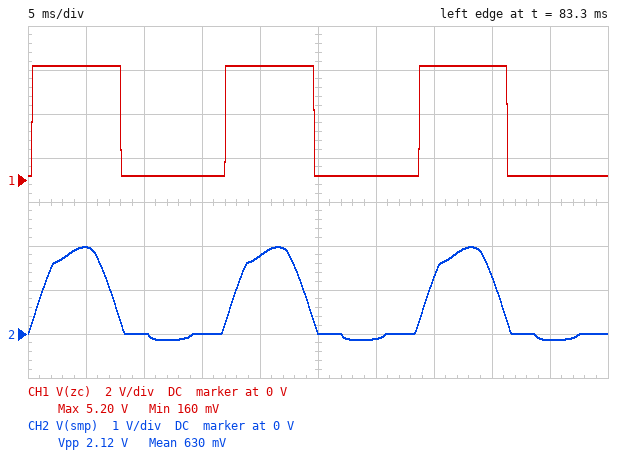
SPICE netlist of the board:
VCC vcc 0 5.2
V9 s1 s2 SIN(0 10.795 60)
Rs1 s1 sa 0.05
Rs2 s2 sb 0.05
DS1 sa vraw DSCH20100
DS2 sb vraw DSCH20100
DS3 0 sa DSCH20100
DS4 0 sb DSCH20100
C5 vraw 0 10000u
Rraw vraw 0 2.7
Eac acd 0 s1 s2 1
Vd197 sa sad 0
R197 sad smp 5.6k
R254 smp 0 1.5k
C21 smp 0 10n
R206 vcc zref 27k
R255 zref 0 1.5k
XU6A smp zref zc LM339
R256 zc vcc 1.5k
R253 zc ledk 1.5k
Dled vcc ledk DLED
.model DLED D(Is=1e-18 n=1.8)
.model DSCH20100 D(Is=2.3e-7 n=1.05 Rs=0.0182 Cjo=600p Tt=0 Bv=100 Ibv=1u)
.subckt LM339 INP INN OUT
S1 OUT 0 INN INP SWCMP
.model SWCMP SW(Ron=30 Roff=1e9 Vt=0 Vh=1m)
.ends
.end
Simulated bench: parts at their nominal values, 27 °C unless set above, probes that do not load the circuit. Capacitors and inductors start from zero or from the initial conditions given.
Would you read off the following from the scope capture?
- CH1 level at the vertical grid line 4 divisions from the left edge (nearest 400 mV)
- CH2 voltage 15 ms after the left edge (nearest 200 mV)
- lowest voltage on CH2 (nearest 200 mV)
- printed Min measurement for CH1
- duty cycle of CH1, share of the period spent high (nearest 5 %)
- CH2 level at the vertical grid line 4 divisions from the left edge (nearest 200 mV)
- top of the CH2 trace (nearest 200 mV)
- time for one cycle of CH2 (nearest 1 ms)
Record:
5.2 V
0 V
-200 mV
160 mV
45 %
1.8 V
2.0 V
17 ms
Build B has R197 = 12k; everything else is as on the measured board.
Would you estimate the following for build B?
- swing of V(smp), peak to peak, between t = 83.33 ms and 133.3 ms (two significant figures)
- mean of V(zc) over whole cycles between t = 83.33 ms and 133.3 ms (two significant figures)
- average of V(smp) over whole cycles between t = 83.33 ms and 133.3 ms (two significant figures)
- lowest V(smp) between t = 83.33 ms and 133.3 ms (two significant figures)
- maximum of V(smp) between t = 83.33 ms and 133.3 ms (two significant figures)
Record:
1.1 V
2.3 V
330 mV
-78 mV
1.0 V
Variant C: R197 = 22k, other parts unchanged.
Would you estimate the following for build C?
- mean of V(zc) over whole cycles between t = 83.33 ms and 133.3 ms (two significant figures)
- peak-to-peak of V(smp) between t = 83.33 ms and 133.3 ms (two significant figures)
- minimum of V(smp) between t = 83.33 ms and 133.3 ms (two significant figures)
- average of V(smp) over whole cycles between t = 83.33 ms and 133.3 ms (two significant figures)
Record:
2.0 V
640 mV
-45 mV
190 mV
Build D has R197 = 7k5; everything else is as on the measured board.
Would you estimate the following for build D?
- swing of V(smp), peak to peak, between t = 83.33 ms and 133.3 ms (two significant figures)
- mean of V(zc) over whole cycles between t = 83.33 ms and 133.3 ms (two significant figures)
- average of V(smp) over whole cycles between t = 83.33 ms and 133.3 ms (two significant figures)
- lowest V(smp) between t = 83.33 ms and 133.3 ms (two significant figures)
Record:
1.7 V
2.4 V
500 mV
-120 mV
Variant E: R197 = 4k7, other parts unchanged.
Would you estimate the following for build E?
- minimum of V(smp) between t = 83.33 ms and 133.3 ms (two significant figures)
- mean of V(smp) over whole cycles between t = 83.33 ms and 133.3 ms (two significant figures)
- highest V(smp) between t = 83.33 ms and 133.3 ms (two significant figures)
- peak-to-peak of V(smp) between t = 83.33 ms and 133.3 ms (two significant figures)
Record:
-170 mV
720 mV
2.3 V
2.4 V
